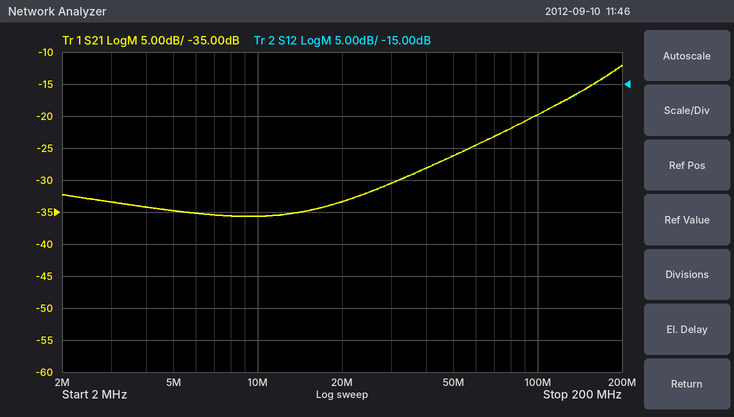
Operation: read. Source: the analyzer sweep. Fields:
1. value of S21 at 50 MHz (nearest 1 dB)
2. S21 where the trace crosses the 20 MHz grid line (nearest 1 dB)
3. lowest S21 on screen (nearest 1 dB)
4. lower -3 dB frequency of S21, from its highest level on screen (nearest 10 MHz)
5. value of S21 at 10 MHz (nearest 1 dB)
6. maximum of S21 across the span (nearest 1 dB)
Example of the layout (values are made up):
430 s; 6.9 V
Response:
-26 dB; -33 dB; -36 dB; 160 MHz; -36 dB; -12 dB
